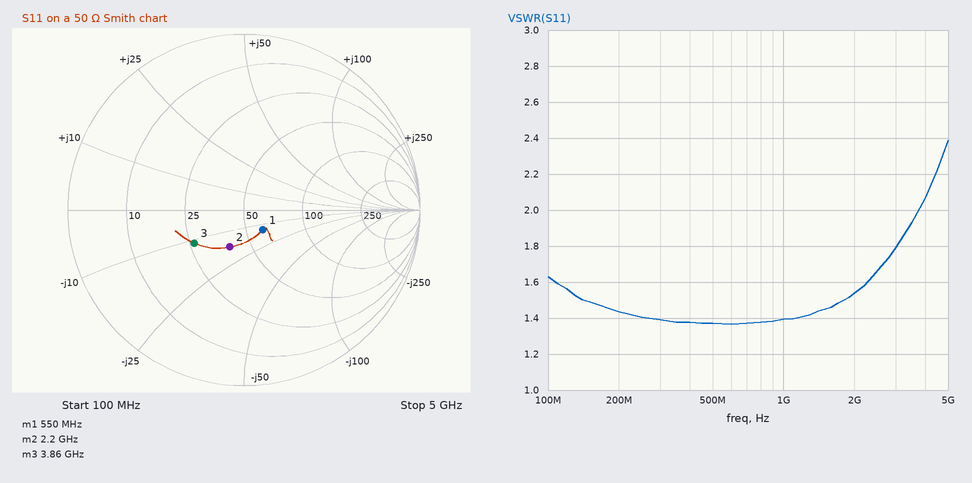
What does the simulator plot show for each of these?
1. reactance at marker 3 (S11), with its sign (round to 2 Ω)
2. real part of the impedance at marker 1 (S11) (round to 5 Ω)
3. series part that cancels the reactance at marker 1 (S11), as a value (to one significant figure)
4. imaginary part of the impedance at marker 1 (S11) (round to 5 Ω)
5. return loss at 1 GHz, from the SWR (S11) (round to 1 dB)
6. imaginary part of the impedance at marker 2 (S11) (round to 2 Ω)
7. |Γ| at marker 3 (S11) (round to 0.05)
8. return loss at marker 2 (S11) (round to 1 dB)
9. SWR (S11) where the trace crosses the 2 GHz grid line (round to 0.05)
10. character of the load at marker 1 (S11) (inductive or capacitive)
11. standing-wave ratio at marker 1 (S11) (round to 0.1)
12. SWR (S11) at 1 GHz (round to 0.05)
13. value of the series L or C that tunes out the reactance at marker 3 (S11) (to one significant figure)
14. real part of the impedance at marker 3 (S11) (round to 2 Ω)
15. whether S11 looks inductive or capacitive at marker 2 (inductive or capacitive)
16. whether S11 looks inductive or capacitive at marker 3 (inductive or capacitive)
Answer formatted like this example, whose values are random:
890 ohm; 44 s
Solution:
-12 Ω; 60 Ω; 4 nH; -15 Ω; 16 dB; -18 Ω; 0.35; 13 dB; 1.55; capacitive; 1.4; 1.40; 500 pH; 26 Ω; capacitive; capacitive
